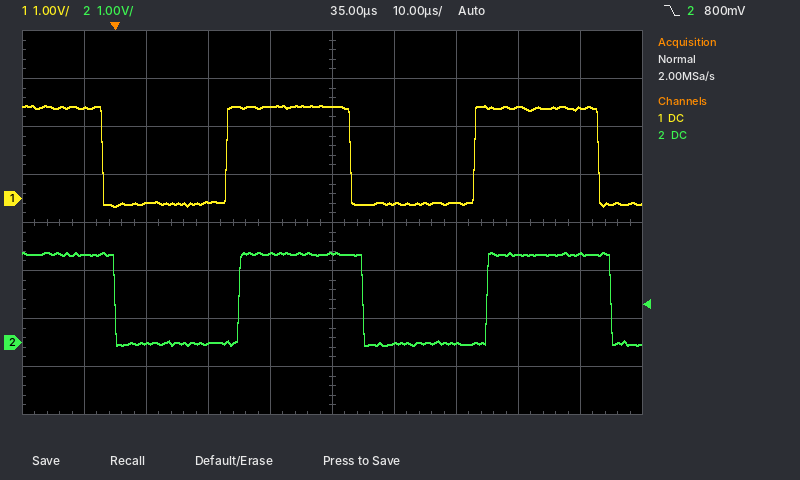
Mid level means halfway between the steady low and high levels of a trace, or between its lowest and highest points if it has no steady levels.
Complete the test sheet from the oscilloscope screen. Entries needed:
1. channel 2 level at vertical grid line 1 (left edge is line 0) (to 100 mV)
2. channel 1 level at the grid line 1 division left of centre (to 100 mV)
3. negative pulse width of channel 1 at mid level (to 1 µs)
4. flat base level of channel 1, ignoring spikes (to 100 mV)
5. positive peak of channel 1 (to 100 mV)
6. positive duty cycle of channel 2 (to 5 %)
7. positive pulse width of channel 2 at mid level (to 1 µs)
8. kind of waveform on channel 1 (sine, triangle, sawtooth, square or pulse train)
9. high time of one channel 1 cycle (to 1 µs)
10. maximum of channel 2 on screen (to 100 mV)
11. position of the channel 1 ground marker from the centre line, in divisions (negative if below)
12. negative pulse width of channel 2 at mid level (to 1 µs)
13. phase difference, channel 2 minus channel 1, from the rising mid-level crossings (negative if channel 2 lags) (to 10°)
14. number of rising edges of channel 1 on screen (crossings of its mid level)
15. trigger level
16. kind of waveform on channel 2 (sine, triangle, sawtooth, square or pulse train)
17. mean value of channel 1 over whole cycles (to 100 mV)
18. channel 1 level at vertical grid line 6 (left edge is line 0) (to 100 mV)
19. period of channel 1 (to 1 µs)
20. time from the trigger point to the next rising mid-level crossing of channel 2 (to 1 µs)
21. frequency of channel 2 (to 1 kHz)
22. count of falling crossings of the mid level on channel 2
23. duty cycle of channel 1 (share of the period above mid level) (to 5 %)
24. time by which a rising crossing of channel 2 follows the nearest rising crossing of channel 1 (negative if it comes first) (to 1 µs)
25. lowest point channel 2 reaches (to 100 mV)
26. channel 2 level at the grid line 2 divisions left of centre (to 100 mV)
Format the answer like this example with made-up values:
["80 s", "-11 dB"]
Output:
["1.8 V", "1.9 V", "20 µs", "-100 mV", "1.9 V", "50 %", "20 µs", "square", "20 µs", "1.9 V", "+0.5 div", "20 µs", "-20°", "2", "800 mV", "square", "900 mV", "-100 mV", "40 µs", "20 µs", "25 kHz", "3", "50 %", "+2 µs", "-100 mV", "0.0 V"]
